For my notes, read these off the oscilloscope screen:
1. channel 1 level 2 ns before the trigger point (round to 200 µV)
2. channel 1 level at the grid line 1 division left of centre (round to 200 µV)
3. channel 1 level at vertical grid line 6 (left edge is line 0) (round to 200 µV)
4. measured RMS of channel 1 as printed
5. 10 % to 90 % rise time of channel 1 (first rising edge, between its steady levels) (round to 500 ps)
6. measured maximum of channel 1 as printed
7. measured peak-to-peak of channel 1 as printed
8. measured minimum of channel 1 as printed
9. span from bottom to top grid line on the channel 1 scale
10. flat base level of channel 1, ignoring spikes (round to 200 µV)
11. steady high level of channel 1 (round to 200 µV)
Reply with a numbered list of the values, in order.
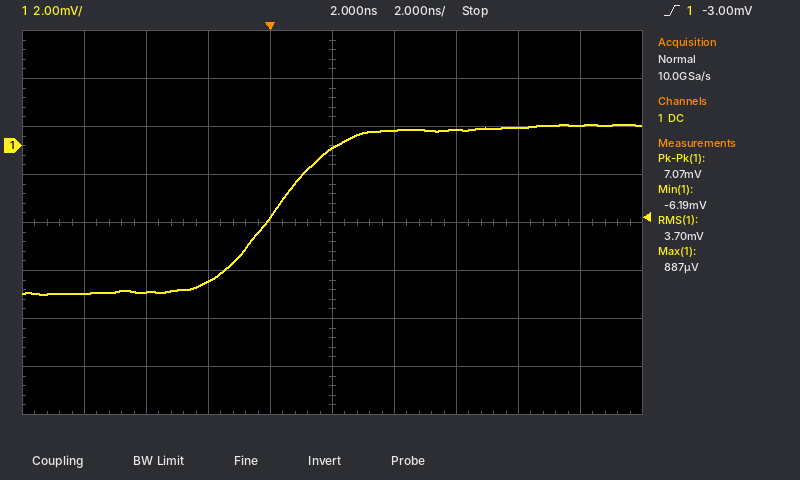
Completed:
1. -5.6 mV
2. -3.0 mV
3. 600 µV
4. 3.70 mV
5. 4.0 ns
6. 887 µV
7. 7.07 mV
8. -6.19 mV
9. 16 mV
10. -6.2 mV
11. 800 µV
